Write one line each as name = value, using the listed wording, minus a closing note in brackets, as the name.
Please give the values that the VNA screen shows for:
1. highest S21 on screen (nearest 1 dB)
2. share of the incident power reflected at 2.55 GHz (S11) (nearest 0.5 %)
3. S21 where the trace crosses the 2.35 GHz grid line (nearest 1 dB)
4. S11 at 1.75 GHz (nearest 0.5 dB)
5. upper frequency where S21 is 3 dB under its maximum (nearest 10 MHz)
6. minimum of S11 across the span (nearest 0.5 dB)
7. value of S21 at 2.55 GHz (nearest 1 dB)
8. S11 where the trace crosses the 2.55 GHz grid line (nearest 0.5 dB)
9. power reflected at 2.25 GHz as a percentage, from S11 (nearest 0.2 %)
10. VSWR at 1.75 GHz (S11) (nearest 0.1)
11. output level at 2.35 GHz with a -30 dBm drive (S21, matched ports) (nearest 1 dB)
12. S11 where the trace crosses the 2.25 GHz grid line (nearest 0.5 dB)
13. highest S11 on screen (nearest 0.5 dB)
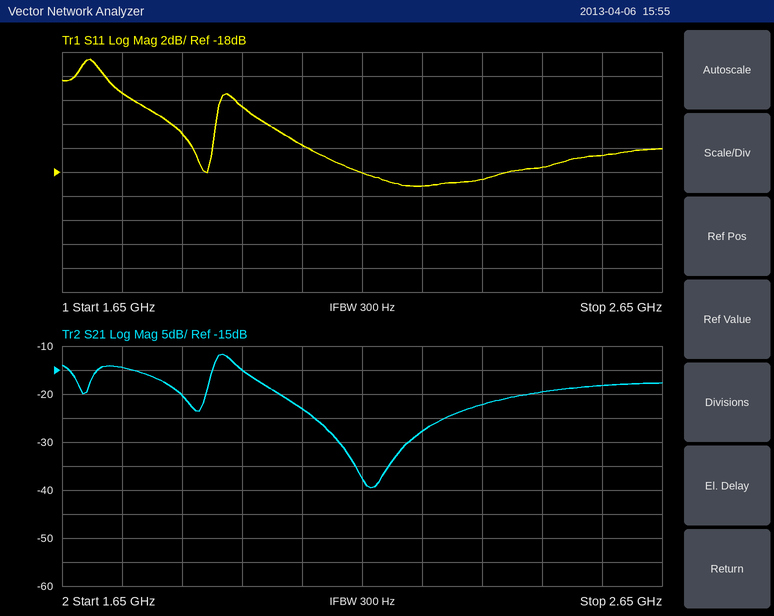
highest S21 on screen = -12 dB
share of the incident power reflected at 2.55 GHz (S11) = 2.0 %
S21 where the trace crosses the 2.35 GHz grid line = -22 dB
S11 at 1.75 GHz = -11.5 dB
upper frequency where S21 is 3 dB under its maximum = 1.95 GHz
minimum of S11 across the span = -19.0 dB
value of S21 at 2.55 GHz = -18 dB
S11 where the trace crosses the 2.55 GHz grid line = -16.5 dB
power reflected at 2.25 GHz as a percentage, from S11 = 1.2 %
VSWR at 1.75 GHz (S11) = 1.7
output level at 2.35 GHz with a -30 dBm drive (S21, matched ports) = -52 dBm
S11 where the trace crosses the 2.25 GHz grid line = -19.0 dB
highest S11 on screen = -8.5 dB
